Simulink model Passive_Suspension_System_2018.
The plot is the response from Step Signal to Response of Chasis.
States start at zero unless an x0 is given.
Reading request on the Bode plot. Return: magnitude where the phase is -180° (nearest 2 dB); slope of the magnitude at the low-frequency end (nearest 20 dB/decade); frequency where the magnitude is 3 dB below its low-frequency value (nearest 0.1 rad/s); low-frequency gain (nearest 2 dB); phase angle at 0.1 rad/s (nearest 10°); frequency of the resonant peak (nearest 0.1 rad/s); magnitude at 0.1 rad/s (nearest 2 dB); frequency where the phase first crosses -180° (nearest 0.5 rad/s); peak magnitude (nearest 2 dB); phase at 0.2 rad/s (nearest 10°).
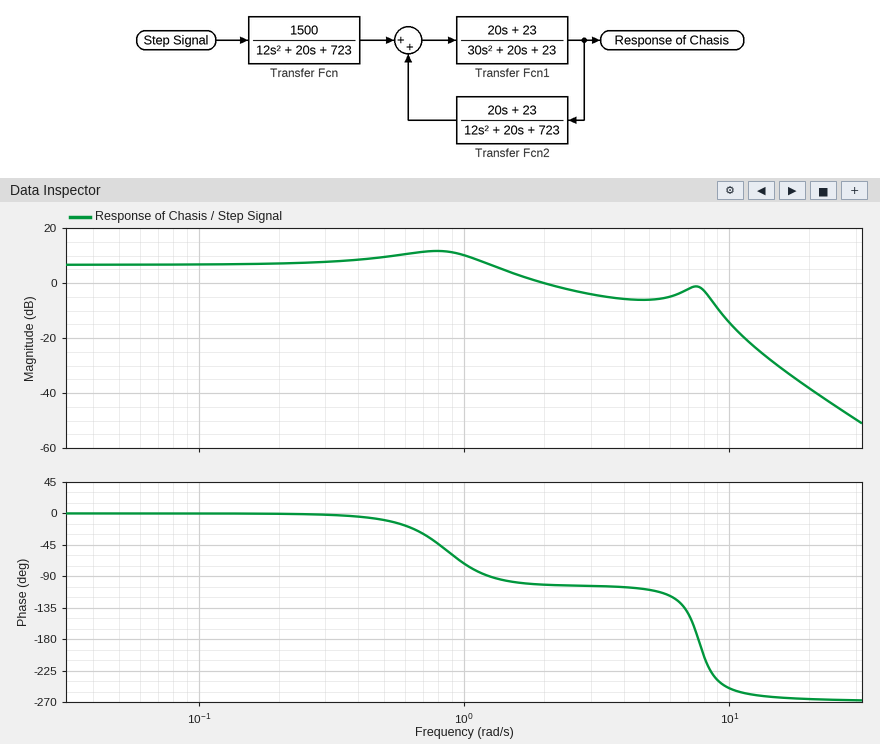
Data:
-2 dB
0 dB/decade
1.5 rad/s
6 dB
0°
0.8 rad/s
6 dB
7.5 rad/s
12 dB
0°
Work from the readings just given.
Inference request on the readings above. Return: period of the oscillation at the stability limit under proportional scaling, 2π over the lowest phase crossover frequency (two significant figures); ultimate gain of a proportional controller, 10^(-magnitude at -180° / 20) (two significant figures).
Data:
0.84 s
1.3
